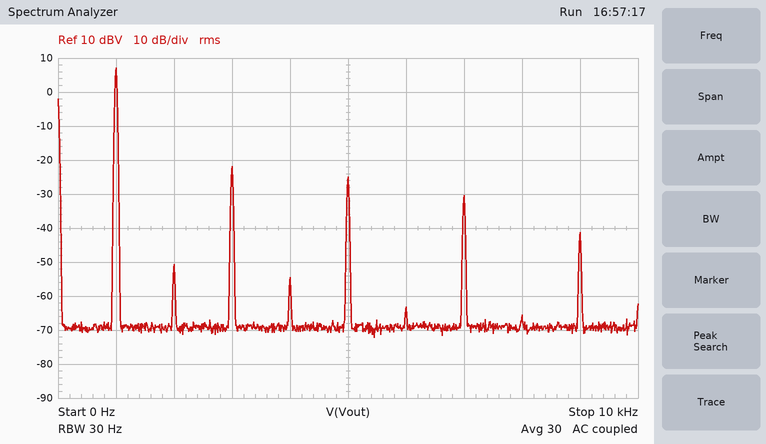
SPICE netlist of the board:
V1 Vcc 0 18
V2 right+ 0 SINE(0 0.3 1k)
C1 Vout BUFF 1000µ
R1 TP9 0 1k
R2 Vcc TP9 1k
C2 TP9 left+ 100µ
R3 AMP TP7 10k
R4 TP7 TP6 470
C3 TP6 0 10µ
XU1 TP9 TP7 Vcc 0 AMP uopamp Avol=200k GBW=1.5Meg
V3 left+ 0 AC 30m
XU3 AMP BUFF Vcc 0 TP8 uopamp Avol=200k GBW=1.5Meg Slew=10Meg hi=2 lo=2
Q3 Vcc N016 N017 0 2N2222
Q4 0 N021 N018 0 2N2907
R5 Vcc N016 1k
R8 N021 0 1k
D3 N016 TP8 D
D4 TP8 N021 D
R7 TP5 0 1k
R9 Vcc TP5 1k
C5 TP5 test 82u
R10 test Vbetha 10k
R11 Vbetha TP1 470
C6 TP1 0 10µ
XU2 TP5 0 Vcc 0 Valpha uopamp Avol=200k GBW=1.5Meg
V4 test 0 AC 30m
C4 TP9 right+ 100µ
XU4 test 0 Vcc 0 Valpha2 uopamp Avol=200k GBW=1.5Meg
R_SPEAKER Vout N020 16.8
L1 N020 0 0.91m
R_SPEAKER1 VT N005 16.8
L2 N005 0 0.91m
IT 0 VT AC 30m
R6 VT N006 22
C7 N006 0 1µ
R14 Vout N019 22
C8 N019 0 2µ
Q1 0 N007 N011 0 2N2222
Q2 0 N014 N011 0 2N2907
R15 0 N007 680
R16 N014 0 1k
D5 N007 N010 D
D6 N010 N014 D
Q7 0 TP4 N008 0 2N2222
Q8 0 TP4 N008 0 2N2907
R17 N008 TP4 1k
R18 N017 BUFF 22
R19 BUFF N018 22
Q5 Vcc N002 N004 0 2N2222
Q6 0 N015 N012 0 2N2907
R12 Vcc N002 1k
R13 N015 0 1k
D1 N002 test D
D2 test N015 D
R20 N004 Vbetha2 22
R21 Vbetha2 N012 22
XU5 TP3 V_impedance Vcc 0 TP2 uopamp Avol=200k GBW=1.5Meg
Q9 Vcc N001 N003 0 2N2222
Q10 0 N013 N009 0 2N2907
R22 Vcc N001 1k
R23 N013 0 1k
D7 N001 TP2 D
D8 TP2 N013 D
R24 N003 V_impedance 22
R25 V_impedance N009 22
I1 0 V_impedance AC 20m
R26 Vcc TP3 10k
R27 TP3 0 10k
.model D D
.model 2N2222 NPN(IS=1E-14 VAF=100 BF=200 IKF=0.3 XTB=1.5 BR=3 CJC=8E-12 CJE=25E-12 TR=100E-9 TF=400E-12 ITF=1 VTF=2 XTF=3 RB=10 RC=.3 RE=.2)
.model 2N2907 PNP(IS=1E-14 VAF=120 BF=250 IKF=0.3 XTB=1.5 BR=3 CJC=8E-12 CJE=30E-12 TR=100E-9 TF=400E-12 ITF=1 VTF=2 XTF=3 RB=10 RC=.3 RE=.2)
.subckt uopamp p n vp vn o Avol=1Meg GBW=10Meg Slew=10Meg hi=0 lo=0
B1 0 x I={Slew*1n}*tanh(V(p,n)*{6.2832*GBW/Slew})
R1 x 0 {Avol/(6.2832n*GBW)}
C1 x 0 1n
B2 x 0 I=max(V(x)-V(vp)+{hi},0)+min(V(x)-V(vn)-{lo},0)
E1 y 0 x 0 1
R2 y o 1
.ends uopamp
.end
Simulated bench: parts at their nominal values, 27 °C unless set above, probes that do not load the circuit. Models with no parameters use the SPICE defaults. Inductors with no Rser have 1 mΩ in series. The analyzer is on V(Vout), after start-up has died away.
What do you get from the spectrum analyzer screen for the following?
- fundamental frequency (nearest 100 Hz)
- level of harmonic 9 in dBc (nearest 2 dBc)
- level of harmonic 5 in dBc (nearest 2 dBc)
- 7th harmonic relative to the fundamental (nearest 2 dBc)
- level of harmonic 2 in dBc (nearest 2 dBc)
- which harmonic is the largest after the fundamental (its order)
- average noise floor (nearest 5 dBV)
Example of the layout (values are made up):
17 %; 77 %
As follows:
1.0 kHz; -48 dBc; -32 dBc; -38 dBc; -58 dBc; 3; -70 dBV
